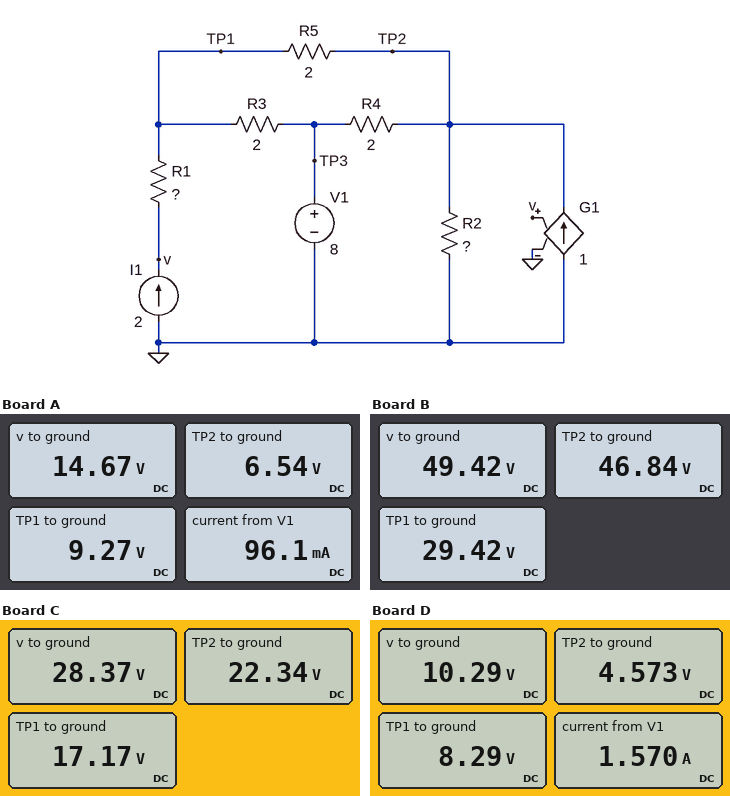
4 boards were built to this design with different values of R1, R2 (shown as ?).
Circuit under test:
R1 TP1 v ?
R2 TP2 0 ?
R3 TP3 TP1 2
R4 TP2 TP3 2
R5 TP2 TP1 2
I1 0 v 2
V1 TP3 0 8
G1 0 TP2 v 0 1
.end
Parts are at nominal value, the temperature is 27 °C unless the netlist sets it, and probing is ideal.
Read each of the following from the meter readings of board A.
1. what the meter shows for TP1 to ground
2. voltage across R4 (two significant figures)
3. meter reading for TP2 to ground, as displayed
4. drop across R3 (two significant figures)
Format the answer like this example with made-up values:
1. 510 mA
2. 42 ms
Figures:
1. 9.27 V
2. 1.5 V
3. 6.54 V
4. 1.3 V
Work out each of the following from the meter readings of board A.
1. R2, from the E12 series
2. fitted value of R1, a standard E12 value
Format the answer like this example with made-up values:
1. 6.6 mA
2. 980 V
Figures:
1. 0.39 Ω
2. 2.7 Ω
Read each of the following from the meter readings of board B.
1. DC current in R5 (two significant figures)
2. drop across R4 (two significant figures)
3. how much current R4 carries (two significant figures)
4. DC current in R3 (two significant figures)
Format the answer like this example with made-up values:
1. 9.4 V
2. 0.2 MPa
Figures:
1. 8.7 A
2. 39 V
3. 19 A
4. 11 A
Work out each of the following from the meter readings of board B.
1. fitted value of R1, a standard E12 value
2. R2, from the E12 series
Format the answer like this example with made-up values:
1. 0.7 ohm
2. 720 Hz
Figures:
1. 10 Ω
2. 2.2 Ω
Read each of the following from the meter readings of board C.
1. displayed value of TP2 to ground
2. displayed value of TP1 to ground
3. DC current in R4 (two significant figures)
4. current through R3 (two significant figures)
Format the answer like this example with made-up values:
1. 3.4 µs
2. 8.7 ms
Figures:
1. 22.34 V
2. 17.17 V
3. 7.2 A
4. 4.6 A
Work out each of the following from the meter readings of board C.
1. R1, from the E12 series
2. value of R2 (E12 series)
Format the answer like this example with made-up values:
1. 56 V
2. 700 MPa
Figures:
1. 5.6 Ω
2. 1.2 Ω
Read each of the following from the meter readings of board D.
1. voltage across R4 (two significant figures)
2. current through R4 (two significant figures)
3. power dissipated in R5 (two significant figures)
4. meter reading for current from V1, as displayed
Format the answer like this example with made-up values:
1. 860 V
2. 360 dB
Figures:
1. 3.4 V
2. 1.7 A
3. 6.9 W
4. 1.570 A
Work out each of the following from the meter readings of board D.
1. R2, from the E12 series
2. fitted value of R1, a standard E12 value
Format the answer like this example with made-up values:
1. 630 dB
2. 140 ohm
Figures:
1. 0.33 Ω
2. 1 Ω
